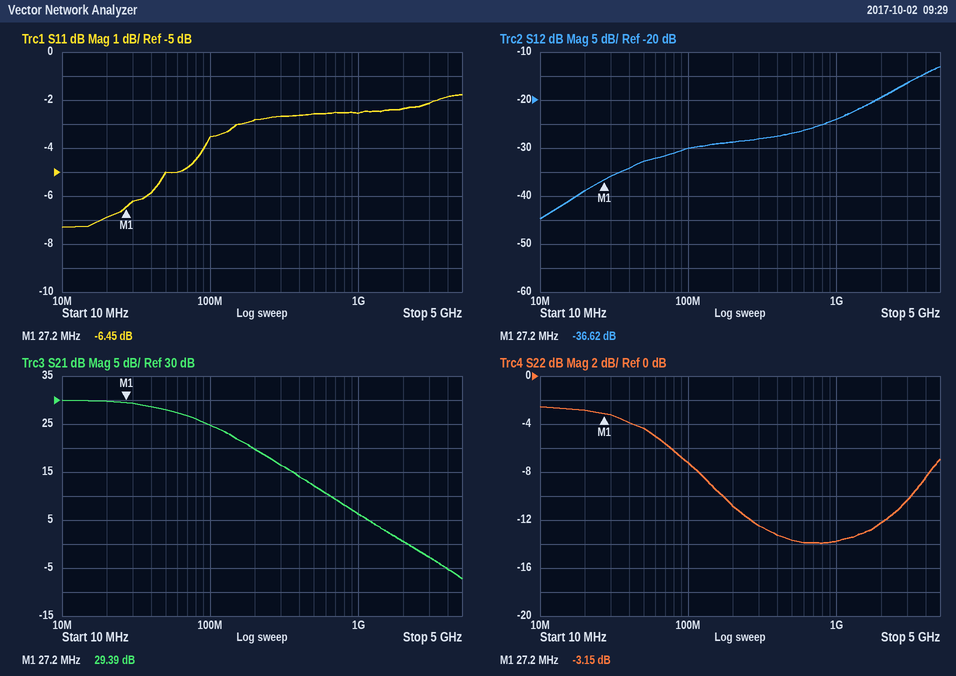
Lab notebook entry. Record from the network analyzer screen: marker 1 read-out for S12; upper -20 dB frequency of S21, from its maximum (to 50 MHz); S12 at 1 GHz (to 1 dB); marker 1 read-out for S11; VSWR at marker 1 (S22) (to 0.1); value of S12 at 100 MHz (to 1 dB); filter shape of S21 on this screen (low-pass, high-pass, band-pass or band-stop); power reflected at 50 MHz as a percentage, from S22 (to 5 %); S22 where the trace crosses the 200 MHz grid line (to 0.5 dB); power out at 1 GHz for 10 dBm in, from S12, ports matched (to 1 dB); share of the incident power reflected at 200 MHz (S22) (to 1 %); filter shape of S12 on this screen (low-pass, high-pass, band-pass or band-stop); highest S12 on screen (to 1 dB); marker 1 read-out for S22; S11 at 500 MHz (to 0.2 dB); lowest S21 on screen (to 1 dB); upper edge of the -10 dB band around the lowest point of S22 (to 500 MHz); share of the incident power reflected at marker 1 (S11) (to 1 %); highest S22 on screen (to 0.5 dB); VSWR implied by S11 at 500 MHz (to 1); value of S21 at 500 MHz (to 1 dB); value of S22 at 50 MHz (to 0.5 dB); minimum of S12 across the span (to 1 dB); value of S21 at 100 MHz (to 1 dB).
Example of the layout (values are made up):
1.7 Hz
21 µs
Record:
-36.62 dB
650 MHz
-24 dB
-6.45 dB
5.6
-30 dB
low-pass
35 %
-11.0 dB
-14 dBm
8 %
high-pass
-13 dB
-3.15 dB
-2.6 dB
-7 dB
3.0 GHz
23 %
-2.5 dB
7
12 dB
-4.5 dB
-45 dB
25 dB
